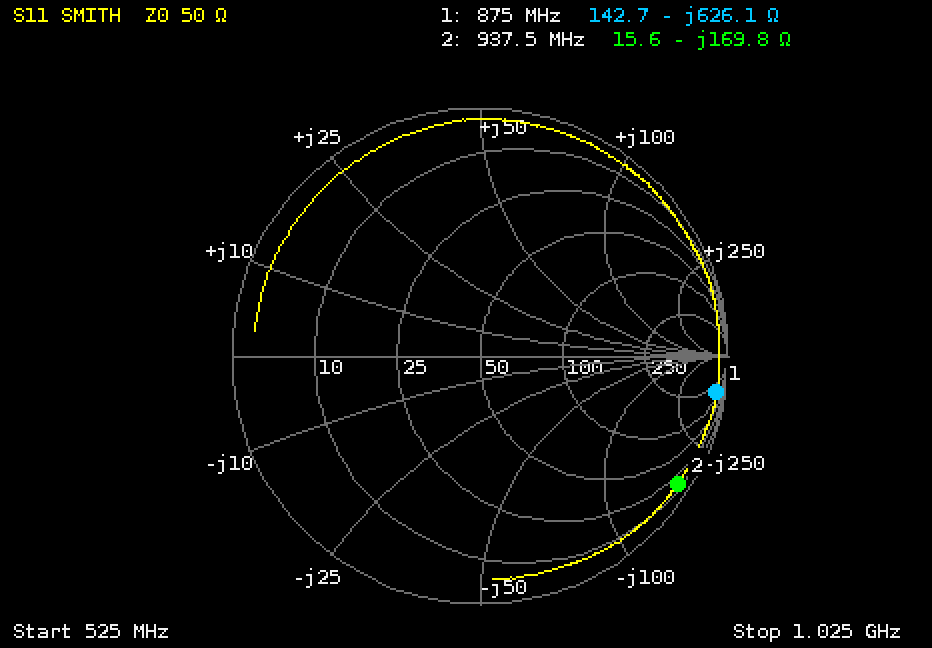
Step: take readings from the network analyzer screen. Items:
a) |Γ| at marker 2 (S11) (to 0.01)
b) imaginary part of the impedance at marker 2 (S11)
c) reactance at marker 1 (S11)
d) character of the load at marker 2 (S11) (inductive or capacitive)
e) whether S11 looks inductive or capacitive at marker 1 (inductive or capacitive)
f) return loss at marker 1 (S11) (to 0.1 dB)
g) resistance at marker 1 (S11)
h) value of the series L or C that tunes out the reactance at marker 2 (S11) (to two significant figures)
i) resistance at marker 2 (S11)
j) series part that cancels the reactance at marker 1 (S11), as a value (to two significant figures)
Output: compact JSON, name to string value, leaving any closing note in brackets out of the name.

{"|Γ| at marker 2 (S11)": "0.95", "imaginary part of the impedance at marker 2": "-169.8 Ω", "reactance at marker 1": "-626.1 Ω", "character of the load at marker 2 (S11)": "capacitive", "whether S11 looks inductive or capacitive at marker 1": "capacitive", "return loss at marker 1 (S11)": "0.3 dB", "resistance at marker 1": "142.7 Ω", "value of the series L or C that tunes out the reactance at marker 2 (S11)": "29 nH", "resistance at marker 2": "15.6 Ω", "series part that cancels the reactance at marker 1 (S11), as a value": "110 nH"}
